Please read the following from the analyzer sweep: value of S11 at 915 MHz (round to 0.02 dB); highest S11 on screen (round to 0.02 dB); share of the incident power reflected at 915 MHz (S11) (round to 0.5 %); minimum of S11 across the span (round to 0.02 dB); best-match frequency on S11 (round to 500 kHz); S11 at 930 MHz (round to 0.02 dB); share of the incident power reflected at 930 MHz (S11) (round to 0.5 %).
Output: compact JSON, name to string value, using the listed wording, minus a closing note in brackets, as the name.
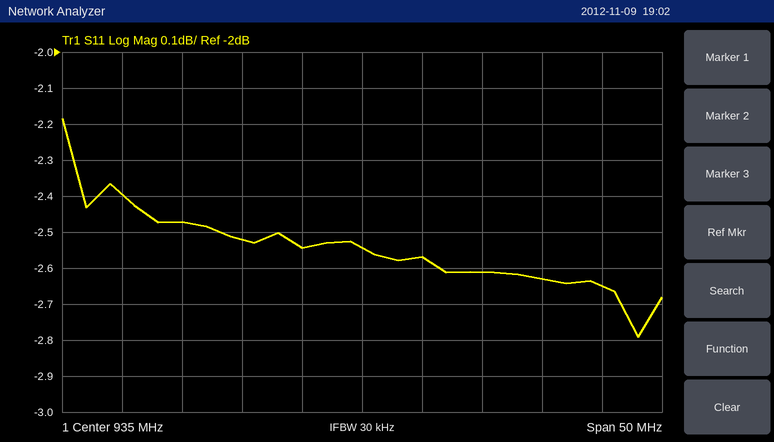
{"value of S11 at 915 MHz": "-2.40 dB", "highest S11 on screen": "-2.18 dB", "share of the incident power reflected at 915 MHz (S11)": "57.5 %", "minimum of S11 across the span": "-2.80 dB", "best-match frequency on S11": "958.0 MHz", "S11 at 930 MHz": "-2.54 dB", "share of the incident power reflected at 930 MHz (S11)": "55.5 %"}
